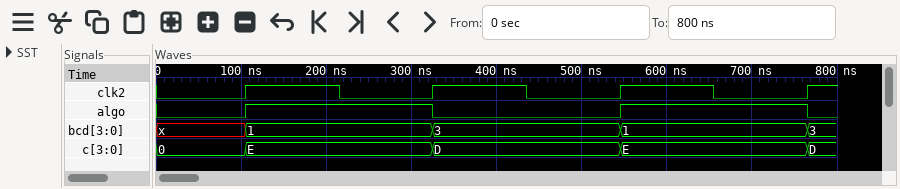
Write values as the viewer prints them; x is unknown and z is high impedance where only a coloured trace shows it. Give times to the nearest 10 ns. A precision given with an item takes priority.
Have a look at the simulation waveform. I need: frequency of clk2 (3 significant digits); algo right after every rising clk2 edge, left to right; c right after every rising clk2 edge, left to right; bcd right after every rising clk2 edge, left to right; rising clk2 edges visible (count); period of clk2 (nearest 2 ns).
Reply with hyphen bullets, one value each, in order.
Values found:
- 4.55 MHz
- 1 0 1 0
- E, D, E, D
- 1, 3, 1, 3
- 4
- 220 ns
